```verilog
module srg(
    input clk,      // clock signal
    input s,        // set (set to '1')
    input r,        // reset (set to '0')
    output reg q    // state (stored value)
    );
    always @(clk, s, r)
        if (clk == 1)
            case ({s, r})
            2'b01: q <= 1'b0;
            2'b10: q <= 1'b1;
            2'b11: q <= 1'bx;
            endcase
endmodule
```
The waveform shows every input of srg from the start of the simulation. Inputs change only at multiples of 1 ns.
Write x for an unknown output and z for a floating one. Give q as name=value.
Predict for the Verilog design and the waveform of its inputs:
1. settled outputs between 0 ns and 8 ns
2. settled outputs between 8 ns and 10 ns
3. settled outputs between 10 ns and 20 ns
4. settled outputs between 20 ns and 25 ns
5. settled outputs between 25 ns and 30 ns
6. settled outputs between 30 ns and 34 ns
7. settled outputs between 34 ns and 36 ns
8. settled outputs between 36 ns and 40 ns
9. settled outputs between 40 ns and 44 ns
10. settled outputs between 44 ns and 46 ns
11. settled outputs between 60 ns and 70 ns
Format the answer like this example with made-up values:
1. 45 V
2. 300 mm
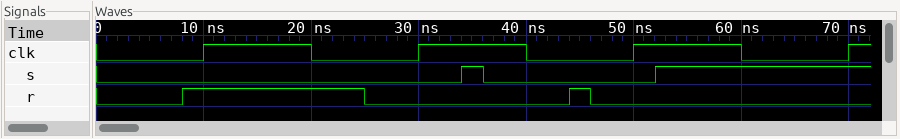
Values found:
1. q=x
2. q=x
3. q=0
4. q=0
5. q=0
6. q=0
7. q=1
8. q=1
9. q=1
10. q=1
11. q=1
